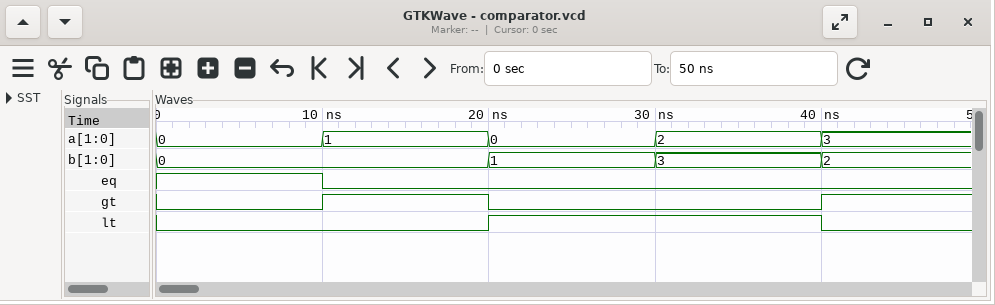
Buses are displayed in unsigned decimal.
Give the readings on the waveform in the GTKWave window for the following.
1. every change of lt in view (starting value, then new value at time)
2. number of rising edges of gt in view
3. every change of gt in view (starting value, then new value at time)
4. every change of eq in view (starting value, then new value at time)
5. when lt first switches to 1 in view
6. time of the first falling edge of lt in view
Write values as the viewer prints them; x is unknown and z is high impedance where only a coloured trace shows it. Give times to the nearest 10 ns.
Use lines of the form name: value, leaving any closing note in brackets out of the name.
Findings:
every change of lt in view: 0, 1 at 20 ns, 0 at 40 ns
number of rising edges of gt in view: 2
every change of gt in view: 0, 1 at 10 ns, 0 at 20 ns, 1 at 40 ns
every change of eq in view: 1, 0 at 10 ns
when lt first switches to 1 in view: 20 ns
time of the first falling edge of lt in view: 40 ns
